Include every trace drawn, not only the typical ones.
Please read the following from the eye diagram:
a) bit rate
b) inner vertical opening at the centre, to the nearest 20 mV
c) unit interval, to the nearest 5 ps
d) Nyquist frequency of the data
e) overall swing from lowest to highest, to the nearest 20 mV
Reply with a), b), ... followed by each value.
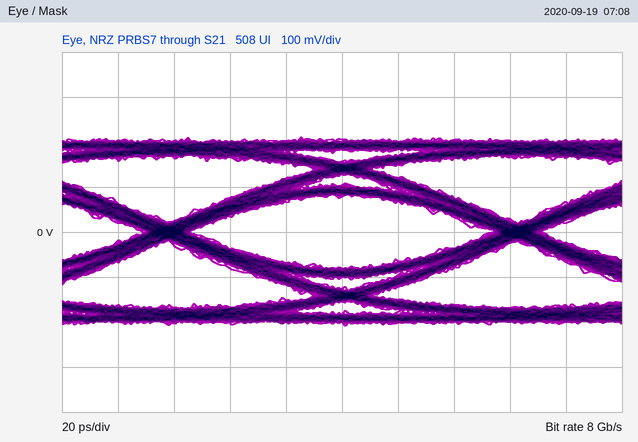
a) 8 Gb/s
b) 160 mV
c) 125 ps
d) 4 GHz
e) 420 mV
